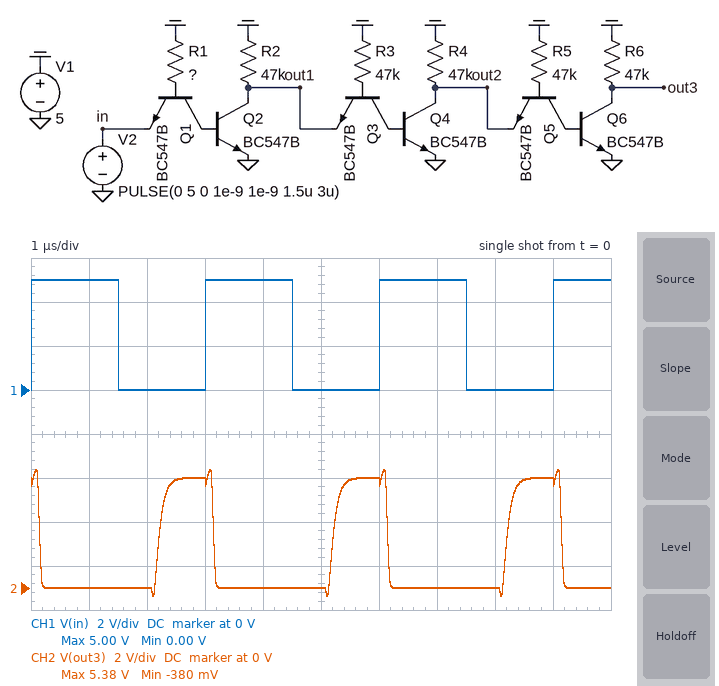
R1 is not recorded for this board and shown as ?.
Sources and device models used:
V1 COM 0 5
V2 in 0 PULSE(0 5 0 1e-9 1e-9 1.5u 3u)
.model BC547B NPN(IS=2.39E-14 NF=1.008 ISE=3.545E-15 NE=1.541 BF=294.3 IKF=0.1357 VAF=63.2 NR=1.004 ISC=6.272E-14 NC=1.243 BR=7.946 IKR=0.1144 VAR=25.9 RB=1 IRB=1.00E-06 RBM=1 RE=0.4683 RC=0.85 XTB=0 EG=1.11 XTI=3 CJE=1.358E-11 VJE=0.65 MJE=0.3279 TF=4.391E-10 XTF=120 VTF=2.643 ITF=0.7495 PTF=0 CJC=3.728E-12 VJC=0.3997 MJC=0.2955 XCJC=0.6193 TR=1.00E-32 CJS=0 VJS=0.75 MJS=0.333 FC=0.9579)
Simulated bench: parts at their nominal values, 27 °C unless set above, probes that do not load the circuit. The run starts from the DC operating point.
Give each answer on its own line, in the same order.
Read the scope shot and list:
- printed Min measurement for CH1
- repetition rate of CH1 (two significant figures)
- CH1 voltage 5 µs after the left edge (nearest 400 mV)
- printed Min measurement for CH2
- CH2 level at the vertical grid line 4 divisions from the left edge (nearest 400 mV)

0.00 V
330 kHz
0 V
-380 mV
0 V
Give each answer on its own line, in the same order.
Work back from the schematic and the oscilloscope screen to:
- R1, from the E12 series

68 kΩ
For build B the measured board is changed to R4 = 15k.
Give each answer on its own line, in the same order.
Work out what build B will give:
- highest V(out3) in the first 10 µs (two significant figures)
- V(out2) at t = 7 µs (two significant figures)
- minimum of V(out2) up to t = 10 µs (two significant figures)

5.4 V
690 mV
-360 mV
